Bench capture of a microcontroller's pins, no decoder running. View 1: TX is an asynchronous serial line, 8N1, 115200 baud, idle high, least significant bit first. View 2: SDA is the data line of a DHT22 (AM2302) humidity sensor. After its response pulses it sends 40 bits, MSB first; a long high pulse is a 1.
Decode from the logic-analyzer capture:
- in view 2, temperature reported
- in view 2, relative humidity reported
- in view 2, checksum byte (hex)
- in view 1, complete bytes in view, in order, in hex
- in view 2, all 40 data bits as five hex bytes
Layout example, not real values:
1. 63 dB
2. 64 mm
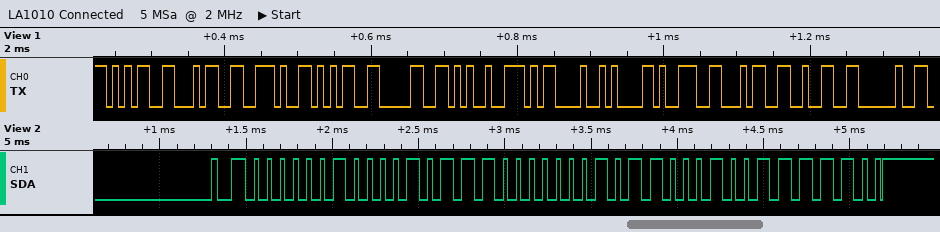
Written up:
1. 35.4 °C
2. 53.5 %
3. 0x7C
4. 35 34 2E 35 30 25 0D 0A 39 34 32 20
5. 02 17 01 62 7C
